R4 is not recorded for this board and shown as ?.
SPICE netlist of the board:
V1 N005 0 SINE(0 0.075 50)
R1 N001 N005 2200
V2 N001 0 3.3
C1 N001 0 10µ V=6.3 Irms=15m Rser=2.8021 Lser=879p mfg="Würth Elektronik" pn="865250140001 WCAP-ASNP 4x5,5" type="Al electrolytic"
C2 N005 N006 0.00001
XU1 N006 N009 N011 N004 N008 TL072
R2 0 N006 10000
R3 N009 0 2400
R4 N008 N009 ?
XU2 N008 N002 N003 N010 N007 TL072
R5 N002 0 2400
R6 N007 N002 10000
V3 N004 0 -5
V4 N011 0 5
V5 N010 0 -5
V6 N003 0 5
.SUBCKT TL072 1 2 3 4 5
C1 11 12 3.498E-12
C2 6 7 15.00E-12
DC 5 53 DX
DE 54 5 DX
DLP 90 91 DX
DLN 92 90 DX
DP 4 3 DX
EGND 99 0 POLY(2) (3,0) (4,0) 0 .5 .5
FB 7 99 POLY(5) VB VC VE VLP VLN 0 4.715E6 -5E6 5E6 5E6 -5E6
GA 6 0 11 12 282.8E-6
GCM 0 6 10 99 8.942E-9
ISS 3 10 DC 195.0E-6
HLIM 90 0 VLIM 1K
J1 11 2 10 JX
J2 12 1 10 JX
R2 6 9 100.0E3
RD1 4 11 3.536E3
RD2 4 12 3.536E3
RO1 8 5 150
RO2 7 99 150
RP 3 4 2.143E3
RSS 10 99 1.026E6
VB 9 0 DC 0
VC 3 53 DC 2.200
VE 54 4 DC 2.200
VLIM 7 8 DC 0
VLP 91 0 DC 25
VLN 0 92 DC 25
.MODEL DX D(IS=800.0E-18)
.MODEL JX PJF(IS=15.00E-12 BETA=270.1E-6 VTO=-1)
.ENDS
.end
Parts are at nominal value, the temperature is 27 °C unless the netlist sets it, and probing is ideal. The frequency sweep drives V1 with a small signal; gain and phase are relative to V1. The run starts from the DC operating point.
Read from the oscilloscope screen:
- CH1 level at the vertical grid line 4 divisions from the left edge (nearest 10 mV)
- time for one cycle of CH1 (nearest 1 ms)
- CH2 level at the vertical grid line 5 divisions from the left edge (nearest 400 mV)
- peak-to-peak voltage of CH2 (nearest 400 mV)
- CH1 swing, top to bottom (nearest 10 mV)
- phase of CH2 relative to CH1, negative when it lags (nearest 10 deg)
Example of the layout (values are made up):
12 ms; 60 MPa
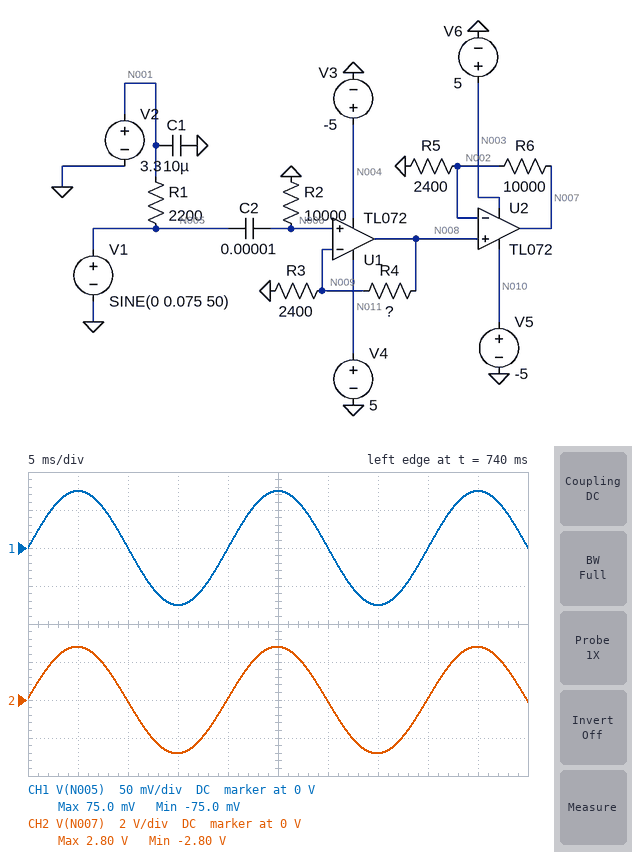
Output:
0 V; 20 ms; 2.8 V; 5.6 V; 150 mV; 0 deg
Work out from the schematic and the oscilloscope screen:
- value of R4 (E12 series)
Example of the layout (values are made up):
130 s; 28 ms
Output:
15 kΩ
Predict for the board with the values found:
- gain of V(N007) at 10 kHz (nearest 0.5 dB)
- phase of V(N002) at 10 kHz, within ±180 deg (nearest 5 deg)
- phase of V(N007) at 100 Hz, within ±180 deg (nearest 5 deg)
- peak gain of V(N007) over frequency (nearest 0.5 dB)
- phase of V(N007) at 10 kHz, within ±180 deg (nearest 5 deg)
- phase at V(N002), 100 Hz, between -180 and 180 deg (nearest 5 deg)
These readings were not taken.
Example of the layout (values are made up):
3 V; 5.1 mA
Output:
31.5 dB; 0 deg; 0 deg; 31.5 dB; 0 deg; 0 deg
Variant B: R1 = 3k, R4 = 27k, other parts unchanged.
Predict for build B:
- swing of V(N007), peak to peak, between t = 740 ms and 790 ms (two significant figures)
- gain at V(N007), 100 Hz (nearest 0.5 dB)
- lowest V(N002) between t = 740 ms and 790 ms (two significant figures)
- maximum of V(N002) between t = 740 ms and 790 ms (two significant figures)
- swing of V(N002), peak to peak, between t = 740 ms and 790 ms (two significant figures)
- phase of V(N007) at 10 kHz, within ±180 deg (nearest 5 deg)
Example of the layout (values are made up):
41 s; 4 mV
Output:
6.9 V; 36.0 dB; -670 mV; 670 mV; 1.3 V; -5 deg
